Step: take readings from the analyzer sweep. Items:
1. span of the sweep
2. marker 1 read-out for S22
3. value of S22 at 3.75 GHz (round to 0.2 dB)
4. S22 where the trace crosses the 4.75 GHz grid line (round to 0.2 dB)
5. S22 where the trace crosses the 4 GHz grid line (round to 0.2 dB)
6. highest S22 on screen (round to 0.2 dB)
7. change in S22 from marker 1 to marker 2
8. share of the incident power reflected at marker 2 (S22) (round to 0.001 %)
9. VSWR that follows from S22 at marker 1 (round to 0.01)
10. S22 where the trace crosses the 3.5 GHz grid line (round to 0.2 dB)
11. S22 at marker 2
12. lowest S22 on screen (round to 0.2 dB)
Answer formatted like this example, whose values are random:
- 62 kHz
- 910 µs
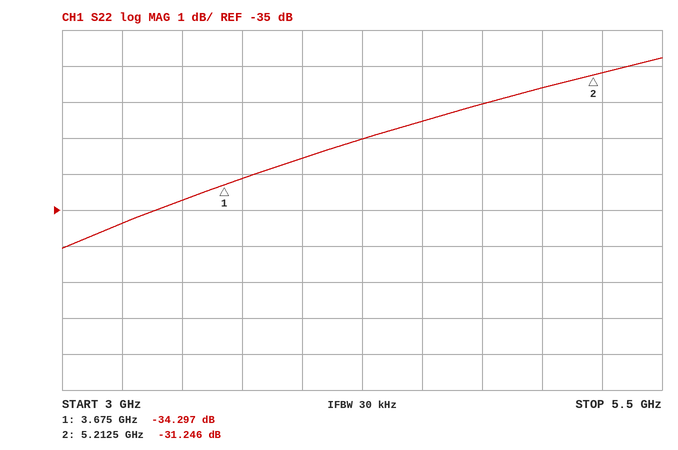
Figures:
- 2.5 GHz
- -34.297 dB
- -34.2 dB
- -32.0 dB
- -33.6 dB
- -30.8 dB
- 3.051 dB
- 0.075 %
- 1.04
- -34.8 dB
- -31.246 dB
- -36.0 dB
